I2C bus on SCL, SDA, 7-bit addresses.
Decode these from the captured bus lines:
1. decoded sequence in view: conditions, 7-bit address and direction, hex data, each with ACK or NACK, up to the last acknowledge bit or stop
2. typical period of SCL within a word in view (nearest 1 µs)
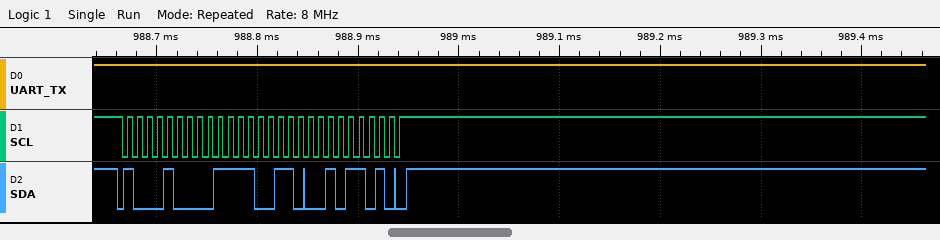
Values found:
start, address 44 write ACK, F3 ACK, 2D ACK, stop
10 µs
